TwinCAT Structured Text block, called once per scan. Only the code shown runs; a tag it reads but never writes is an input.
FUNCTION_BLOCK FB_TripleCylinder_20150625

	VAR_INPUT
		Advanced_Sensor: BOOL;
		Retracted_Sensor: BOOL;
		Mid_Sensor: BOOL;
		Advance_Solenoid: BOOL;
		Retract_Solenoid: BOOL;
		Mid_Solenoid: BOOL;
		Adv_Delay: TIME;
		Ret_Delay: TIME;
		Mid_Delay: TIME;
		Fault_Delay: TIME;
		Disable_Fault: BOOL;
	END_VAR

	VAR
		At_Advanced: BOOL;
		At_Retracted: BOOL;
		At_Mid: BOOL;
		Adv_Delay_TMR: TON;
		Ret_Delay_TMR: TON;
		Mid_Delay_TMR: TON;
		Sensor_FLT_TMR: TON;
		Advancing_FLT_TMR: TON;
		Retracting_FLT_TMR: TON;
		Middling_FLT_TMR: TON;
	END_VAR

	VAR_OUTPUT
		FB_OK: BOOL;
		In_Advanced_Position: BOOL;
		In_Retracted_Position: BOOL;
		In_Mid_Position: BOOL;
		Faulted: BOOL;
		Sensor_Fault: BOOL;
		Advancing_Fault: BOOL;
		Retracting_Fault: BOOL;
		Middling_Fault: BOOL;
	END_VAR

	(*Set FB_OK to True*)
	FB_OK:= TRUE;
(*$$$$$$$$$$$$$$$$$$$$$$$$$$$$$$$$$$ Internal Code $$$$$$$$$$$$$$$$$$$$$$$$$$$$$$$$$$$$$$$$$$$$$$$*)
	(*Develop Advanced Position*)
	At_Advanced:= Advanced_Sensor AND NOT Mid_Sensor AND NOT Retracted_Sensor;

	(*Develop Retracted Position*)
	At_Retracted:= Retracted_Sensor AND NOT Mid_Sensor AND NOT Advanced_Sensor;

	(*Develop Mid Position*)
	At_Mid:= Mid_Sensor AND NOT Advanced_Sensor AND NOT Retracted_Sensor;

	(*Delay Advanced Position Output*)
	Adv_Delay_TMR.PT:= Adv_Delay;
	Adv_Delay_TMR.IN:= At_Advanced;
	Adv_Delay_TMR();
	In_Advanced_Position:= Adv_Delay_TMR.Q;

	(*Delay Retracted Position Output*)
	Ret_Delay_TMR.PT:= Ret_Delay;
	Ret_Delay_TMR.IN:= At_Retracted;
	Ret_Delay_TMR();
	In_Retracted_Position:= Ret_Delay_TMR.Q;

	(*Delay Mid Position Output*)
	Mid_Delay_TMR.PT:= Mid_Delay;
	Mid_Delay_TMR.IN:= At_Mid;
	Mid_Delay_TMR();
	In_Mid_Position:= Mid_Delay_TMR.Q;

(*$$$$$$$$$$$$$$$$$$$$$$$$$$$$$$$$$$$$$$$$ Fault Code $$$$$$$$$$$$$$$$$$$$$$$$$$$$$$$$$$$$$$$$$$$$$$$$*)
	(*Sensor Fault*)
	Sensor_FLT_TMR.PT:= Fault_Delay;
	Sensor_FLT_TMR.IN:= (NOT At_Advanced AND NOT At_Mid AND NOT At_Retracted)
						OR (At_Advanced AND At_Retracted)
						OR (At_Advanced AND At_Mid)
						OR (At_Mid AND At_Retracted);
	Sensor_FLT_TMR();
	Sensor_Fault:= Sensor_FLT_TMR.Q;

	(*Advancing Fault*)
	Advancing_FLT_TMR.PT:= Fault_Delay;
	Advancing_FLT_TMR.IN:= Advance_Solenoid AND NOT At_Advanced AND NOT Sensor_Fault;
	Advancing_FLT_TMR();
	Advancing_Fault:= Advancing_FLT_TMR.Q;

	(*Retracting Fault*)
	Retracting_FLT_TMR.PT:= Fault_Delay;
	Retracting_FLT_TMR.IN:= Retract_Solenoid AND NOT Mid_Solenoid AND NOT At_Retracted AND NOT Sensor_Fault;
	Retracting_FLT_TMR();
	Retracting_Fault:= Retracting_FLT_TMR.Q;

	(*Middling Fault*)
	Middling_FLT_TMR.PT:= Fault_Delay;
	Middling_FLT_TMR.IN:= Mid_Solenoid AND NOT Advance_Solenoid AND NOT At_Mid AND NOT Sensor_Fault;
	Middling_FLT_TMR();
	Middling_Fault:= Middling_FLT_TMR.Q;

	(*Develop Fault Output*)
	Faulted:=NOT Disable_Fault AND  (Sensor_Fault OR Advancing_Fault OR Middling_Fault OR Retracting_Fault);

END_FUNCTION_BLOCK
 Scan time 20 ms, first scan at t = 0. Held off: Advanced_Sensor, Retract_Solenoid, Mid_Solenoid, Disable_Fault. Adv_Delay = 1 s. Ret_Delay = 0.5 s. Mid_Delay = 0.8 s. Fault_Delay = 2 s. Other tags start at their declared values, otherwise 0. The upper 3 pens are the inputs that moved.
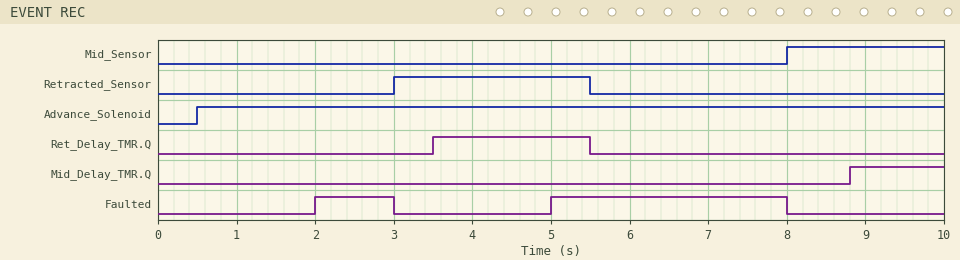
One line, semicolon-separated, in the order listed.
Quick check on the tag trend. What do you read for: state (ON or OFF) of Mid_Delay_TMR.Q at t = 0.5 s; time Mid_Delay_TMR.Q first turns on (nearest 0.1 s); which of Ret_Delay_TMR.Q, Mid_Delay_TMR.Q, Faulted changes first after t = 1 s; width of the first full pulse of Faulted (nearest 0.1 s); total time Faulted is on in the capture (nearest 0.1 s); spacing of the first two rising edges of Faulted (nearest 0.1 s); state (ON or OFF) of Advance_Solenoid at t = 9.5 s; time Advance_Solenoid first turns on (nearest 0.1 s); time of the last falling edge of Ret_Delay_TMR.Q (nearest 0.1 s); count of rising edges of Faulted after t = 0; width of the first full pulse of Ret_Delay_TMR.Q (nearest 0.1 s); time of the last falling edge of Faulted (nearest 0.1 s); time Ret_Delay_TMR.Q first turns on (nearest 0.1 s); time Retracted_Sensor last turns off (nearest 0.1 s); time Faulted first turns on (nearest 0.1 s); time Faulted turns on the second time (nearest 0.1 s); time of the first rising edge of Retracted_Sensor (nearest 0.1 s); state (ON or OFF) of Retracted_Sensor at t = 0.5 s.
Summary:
OFF; 8.8 s; Faulted; 1.0 s; 4.0 s; 3.0 s; ON; 0.5 s; 5.5 s; 2; 2.0 s; 8.0 s; 3.5 s; 5.5 s; 2.0 s; 5.0 s; 3.0 s; OFF
